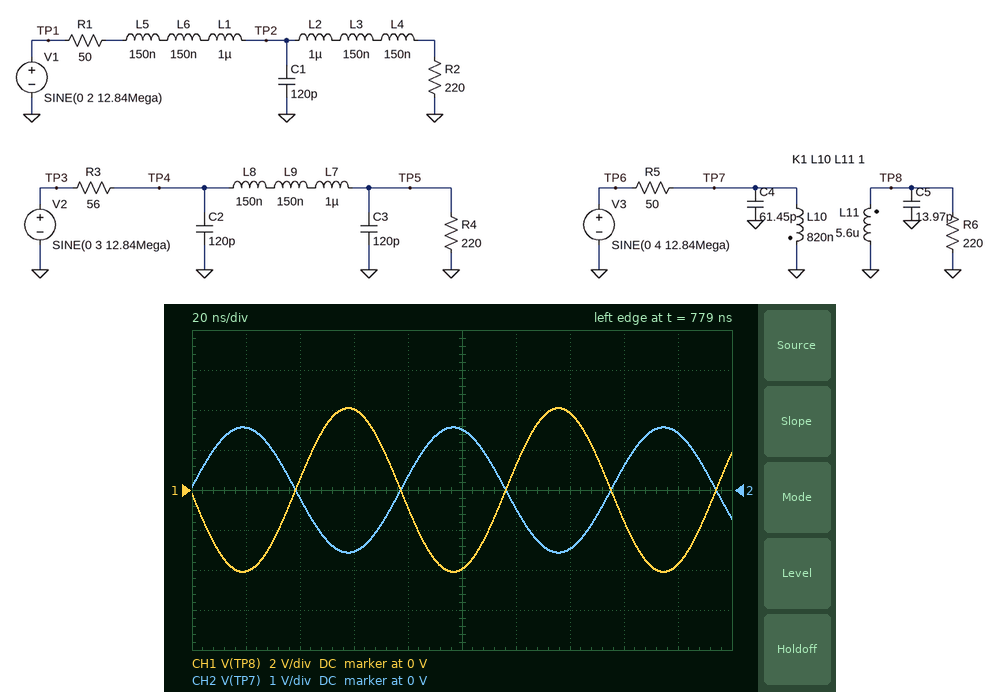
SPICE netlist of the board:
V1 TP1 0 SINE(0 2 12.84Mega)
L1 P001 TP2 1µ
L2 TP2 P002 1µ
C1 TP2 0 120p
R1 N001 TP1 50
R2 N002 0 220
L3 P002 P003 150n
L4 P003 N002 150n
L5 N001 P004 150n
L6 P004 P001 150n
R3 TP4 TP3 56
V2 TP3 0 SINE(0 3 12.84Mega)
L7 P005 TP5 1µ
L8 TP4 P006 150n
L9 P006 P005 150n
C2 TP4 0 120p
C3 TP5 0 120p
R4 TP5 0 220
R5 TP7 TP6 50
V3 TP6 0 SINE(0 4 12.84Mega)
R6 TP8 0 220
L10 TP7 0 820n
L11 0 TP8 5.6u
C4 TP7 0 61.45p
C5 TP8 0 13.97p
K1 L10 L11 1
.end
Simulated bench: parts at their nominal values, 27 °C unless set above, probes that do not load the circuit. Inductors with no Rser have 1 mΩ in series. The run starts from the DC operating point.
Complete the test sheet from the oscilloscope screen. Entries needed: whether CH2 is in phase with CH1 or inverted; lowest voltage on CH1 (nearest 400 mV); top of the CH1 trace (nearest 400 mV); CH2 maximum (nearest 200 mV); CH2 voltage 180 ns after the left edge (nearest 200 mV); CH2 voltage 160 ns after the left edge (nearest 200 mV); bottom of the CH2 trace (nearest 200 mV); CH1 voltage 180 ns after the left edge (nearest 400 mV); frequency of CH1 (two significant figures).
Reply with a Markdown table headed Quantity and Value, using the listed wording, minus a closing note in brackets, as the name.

| Quantity | Value |
|---|---|
| whether CH2 is in phase with CH1 or inverted | inverted |
| lowest voltage on CH1 | -4.0 V |
| top of the CH1 trace | 4.0 V |
| CH2 maximum | 1.6 V |
| CH2 voltage 180 ns after the left edge | 1.4 V |
| CH2 voltage 160 ns after the left edge | 600 mV |
| bottom of the CH2 trace | -1.6 V |
| CH1 voltage 180 ns after the left edge | -3.6 V |
| frequency of CH1 | 13 MHz |
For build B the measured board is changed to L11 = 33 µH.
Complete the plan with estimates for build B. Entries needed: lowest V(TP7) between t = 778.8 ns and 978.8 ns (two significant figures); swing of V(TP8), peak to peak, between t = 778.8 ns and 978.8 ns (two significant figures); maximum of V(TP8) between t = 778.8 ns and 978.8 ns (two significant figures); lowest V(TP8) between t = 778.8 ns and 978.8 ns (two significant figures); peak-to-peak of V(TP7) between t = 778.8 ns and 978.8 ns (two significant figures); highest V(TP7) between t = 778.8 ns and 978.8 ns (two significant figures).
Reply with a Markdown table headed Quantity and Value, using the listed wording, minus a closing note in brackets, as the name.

| Quantity | Value |
|---|---|
| lowest V(TP7) between t = 778.8 ns and 978.8 ns | -390 mV |
| swing of V(TP8), peak to peak, between t = 778.8 ns and 978.8 ns | 4.9 V |
| maximum of V(TP8) between t = 778.8 ns and 978.8 ns | 2.5 V |
| lowest V(TP8) between t = 778.8 ns and 978.8 ns | -2.5 V |
| peak-to-peak of V(TP7) between t = 778.8 ns and 978.8 ns | 780 mV |
| highest V(TP7) between t = 778.8 ns and 978.8 ns | 390 mV |
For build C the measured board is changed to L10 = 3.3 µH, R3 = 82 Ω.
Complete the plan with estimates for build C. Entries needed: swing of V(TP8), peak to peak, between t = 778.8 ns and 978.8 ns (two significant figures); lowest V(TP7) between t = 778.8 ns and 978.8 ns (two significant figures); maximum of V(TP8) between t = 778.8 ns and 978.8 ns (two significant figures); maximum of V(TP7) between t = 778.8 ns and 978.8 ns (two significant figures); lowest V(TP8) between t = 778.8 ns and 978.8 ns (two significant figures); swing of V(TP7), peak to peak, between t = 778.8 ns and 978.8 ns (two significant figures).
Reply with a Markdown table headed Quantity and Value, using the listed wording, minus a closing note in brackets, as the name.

| Quantity | Value |
|---|---|
| swing of V(TP8), peak to peak, between t = 778.8 ns and 978.8 ns | 7.5 V |
| lowest V(TP7) between t = 778.8 ns and 978.8 ns | -2.9 V |
| maximum of V(TP8) between t = 778.8 ns and 978.8 ns | 3.7 V |
| maximum of V(TP7) between t = 778.8 ns and 978.8 ns | 2.9 V |
| lowest V(TP8) between t = 778.8 ns and 978.8 ns | -3.7 V |
| swing of V(TP7), peak to peak, between t = 778.8 ns and 978.8 ns | 5.7 V |
